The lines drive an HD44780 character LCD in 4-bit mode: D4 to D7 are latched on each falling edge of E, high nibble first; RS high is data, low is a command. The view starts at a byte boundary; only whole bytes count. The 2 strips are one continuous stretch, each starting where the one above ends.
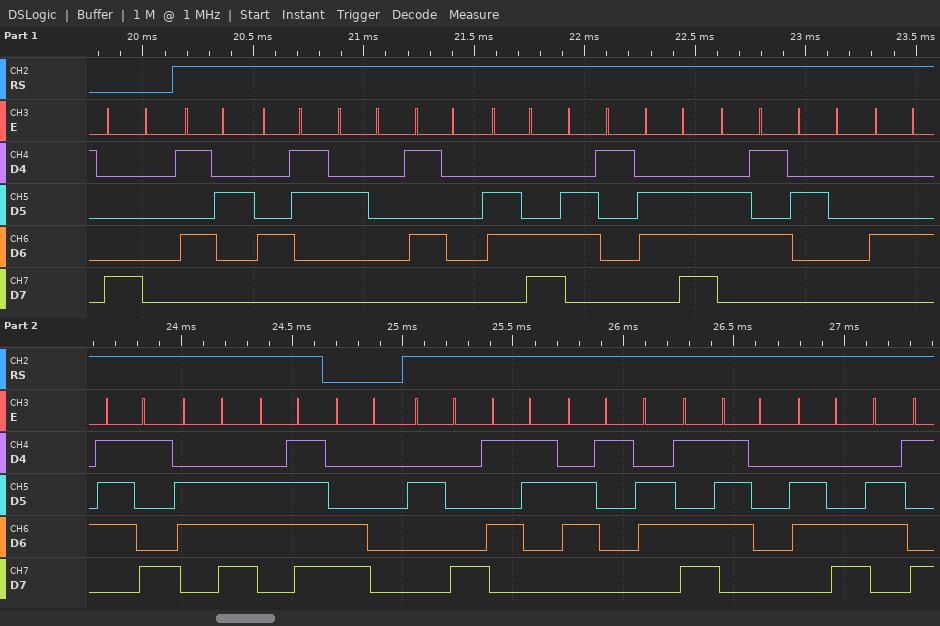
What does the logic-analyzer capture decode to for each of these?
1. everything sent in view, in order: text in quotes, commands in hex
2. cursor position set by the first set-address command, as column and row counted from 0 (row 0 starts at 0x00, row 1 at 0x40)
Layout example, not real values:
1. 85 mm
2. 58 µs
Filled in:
1. 0x80 "RC Plane Dyno" 0xC0 "(Sampli"
2. column 0, row 0
